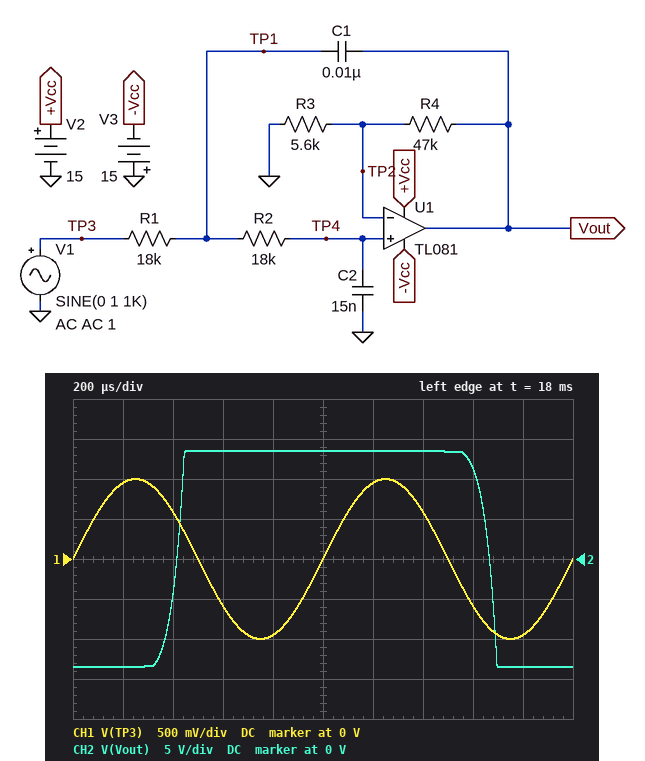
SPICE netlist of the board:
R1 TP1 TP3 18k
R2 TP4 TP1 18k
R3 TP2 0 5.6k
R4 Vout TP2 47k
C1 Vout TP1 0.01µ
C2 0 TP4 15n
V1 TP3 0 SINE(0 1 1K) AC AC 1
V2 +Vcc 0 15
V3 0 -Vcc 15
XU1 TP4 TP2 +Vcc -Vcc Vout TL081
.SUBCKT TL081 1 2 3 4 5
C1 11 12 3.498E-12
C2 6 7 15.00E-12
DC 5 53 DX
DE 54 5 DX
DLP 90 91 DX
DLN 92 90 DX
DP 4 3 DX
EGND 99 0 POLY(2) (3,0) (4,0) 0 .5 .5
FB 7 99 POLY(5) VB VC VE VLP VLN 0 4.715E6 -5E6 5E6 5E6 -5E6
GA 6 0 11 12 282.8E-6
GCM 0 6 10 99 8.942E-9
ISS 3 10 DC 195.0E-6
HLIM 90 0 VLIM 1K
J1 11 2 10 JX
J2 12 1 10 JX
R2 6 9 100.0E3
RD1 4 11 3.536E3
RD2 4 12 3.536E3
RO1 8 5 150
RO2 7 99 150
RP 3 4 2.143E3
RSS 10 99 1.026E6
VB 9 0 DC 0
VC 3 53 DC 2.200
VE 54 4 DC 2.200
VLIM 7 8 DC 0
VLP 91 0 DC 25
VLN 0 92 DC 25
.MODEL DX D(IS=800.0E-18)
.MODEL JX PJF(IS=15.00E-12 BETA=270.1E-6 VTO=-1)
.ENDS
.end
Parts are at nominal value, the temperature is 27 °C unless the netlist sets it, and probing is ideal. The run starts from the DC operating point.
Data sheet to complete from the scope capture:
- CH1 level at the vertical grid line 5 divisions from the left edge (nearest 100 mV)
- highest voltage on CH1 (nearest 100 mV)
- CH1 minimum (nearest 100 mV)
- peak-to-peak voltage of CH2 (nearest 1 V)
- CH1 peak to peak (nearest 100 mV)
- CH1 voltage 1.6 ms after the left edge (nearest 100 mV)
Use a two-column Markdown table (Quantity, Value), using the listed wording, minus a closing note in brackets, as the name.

| Quantity | Value |
|---|---|
| CH1 level at the vertical grid line 5 divisions from the left edge | 0 V |
| highest voltage on CH1 | 1.0 V |
| CH1 minimum | -1.0 V |
| peak-to-peak voltage of CH2 | 27 V |
| CH1 peak to peak | 2.0 V |
| CH1 voltage 1.6 ms after the left edge | -600 mV |
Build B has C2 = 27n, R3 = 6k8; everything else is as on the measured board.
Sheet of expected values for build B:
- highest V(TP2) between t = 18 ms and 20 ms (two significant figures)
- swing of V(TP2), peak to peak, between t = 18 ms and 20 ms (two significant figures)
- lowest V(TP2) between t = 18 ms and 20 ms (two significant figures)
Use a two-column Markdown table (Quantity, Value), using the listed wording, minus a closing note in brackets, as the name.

| Quantity | Value |
|---|---|
| highest V(TP2) between t = 18 ms and 20 ms | 1.7 V |
| swing of V(TP2), peak to peak, between t = 18 ms and 20 ms | 3.4 V |
| lowest V(TP2) between t = 18 ms and 20 ms | -1.7 V |
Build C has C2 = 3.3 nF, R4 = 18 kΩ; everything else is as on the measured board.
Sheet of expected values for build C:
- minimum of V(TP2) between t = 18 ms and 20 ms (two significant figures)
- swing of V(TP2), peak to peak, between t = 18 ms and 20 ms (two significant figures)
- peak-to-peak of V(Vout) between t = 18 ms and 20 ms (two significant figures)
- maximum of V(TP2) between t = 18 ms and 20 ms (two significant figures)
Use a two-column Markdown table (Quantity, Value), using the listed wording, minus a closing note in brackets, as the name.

| Quantity | Value |
|---|---|
| minimum of V(TP2) between t = 18 ms and 20 ms | -3.2 V |
| swing of V(TP2), peak to peak, between t = 18 ms and 20 ms | 6.4 V |
| peak-to-peak of V(Vout) between t = 18 ms and 20 ms | 27 V |
| maximum of V(TP2) between t = 18 ms and 20 ms | 3.2 V |
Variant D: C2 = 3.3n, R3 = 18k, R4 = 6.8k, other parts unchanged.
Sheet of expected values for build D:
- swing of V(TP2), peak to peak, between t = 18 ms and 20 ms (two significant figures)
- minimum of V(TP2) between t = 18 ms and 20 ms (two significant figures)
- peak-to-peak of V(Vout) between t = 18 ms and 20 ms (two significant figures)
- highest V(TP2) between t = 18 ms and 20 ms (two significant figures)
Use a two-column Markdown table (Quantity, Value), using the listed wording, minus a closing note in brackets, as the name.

| Quantity | Value |
|---|---|
| swing of V(TP2), peak to peak, between t = 18 ms and 20 ms | 3.0 V |
| minimum of V(TP2) between t = 18 ms and 20 ms | -1.5 V |
| peak-to-peak of V(Vout) between t = 18 ms and 20 ms | 4.2 V |
| highest V(TP2) between t = 18 ms and 20 ms | 1.5 V |
